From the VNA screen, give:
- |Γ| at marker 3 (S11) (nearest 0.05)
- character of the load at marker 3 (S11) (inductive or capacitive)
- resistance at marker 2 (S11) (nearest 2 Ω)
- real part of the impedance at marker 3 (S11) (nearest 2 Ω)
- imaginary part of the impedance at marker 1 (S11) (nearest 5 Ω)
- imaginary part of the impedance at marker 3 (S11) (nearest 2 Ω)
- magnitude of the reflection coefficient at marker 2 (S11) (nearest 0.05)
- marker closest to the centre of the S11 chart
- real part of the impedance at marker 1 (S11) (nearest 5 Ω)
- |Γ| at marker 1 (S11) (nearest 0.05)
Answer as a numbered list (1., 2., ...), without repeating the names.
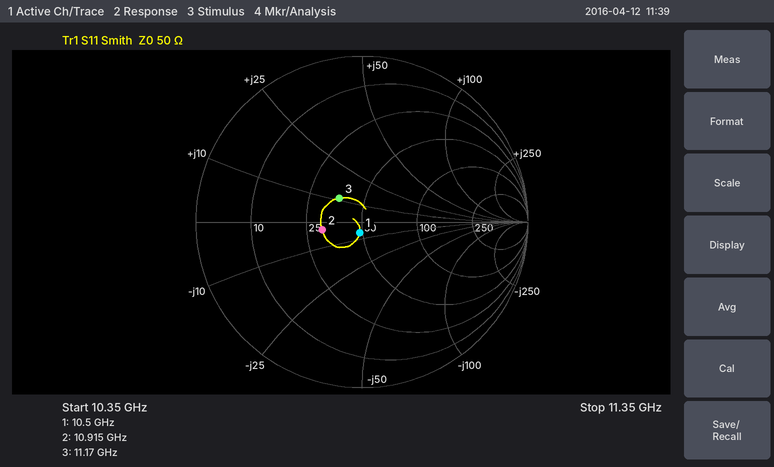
1. 0.20
2. inductive
3. 30 Ω
4. 36 Ω
5. -5 Ω
6. +10 Ω
7. 0.25
8. marker 1
9. 50 Ω
10. 0.05
